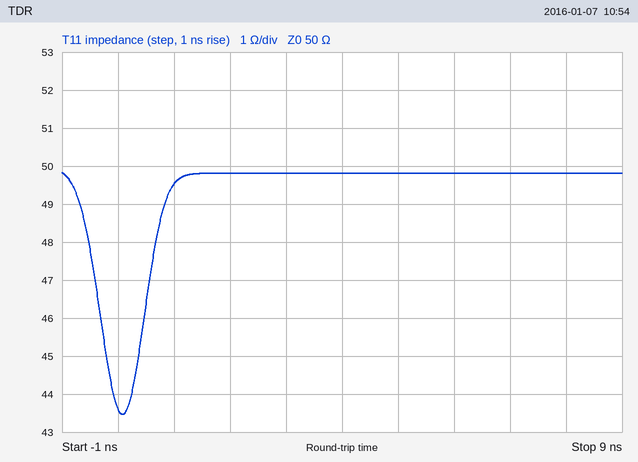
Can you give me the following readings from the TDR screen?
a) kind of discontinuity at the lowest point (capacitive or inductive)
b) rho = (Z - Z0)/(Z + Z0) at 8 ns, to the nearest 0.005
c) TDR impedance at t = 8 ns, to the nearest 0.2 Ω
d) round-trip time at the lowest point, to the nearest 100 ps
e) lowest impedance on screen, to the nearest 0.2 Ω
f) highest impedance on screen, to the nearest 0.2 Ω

capacitive
0.000
49.8 Ω
100 ps
43.4 Ω
49.8 Ω
